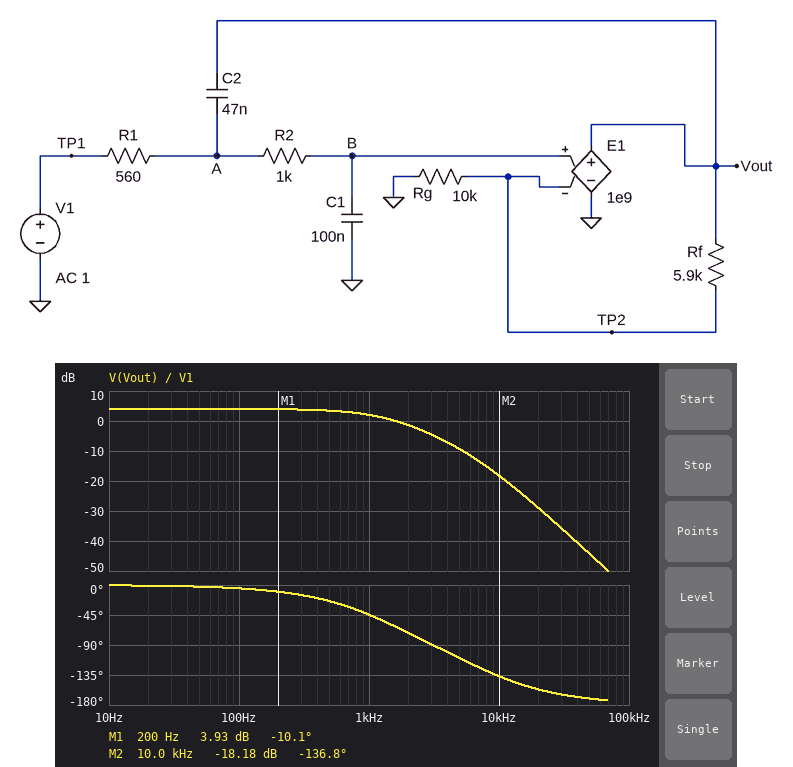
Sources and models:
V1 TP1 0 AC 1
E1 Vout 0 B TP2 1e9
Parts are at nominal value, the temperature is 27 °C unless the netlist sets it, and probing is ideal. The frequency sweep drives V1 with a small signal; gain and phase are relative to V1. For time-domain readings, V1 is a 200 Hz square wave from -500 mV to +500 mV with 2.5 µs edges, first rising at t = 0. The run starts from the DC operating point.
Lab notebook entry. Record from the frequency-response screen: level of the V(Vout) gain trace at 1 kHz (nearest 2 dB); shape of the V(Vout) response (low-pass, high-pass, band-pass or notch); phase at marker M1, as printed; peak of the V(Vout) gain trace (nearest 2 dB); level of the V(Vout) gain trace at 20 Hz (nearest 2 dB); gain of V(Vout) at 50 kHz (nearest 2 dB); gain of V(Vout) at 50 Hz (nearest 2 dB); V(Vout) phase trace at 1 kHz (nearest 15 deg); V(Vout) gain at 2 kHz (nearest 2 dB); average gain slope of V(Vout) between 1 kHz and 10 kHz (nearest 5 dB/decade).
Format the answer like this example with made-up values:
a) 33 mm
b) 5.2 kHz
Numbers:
a) 2 dB
b) low-pass
c) -10.1 deg
d) 4 dB
e) 4 dB
f) -44 dB
g) 4 dB
h) -45 deg
i) -2 dB
j) -20 dB/decade
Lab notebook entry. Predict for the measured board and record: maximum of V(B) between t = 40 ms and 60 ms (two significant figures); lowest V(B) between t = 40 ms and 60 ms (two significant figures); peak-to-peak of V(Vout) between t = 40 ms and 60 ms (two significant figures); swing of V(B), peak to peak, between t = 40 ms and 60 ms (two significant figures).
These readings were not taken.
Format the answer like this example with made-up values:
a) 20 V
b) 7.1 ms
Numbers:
a) 500 mV
b) -500 mV
c) 1.6 V
d) 1.0 V
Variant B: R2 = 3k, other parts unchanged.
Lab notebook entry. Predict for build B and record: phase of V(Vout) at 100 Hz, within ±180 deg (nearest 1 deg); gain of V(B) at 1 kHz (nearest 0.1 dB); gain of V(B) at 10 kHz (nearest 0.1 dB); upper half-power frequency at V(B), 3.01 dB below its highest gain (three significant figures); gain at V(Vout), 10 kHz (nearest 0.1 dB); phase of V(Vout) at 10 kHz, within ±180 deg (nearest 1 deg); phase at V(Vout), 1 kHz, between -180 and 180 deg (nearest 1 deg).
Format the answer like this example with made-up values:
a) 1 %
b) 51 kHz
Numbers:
a) -12 deg
b) -7.0 dB
c) -31.4 dB
d) 501 Hz
e) -27.3 dB
f) -145 deg
g) -72 deg
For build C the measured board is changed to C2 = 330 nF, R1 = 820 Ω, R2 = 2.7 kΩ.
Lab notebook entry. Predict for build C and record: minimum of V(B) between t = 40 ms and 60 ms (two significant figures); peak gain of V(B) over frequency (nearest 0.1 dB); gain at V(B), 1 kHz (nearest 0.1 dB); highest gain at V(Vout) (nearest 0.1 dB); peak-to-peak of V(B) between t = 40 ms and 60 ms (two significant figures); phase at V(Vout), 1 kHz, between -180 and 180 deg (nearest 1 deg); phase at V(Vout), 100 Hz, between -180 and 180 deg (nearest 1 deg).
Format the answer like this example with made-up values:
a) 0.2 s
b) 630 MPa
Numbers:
a) -810 mV
b) 3.5 dB
c) -7.0 dB
d) 7.6 dB
e) 1.6 V
f) -147 deg
g) -7 deg
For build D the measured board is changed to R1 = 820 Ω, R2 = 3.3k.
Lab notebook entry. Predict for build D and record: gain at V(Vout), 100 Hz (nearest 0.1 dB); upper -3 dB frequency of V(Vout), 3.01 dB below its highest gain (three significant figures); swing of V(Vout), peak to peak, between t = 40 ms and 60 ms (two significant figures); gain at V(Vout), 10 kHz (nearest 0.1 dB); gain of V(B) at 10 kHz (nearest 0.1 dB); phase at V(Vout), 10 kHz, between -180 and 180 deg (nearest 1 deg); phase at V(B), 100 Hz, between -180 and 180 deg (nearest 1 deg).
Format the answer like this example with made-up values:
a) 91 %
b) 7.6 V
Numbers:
a) 3.8 dB
b) 446 Hz
c) 1.6 V
d) -30.8 dB
e) -34.8 dB
f) -154 deg
g) -14 deg
